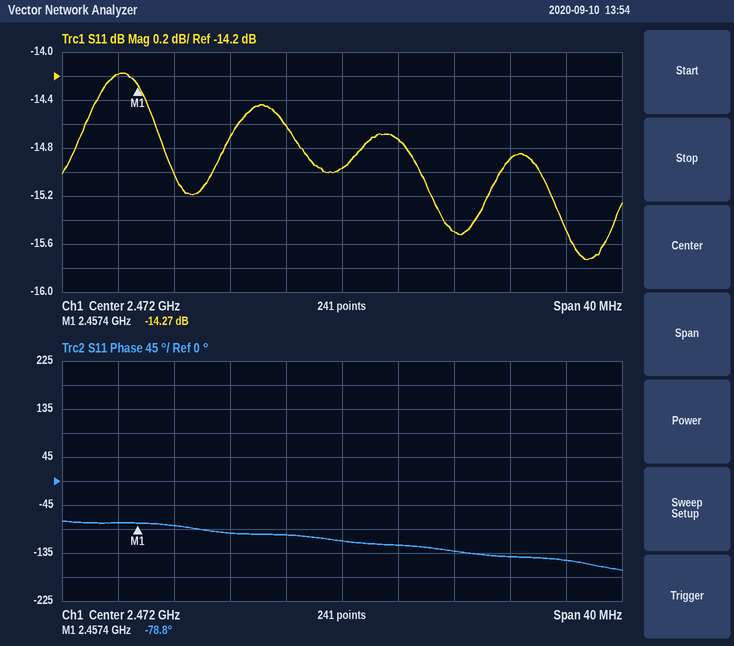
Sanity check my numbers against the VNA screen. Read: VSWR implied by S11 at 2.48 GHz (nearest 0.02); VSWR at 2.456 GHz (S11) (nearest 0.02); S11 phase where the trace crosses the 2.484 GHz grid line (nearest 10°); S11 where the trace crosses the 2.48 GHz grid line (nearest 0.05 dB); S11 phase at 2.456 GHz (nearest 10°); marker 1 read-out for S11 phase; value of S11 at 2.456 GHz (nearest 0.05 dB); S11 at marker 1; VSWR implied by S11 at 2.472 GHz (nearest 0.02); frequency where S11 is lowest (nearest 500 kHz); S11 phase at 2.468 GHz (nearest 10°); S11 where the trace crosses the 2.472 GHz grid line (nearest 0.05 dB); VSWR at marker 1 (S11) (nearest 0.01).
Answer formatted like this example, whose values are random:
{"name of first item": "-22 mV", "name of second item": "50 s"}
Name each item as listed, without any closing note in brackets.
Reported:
{"VSWR implied by S11 at 2.48 GHz": "1.40", "VSWR at 2.456 GHz (S11)": "1.48", "S11 phase where the trace crosses the 2.484 GHz grid line": "-140°", "S11 where the trace crosses the 2.48 GHz grid line": "-15.50 dB", "S11 phase at 2.456 GHz": "-80°", "marker 1 read-out for S11 phase": "-78.8°", "value of S11 at 2.456 GHz": "-14.20 dB", "S11 at marker 1": "-14.27 dB", "VSWR implied by S11 at 2.472 GHz": "1.44", "frequency where S11 is lowest": "2.4895 GHz", "S11 phase at 2.468 GHz": "-100°", "S11 where the trace crosses the 2.472 GHz grid line": "-14.95 dB", "VSWR at marker 1 (S11)": "1.48"}
